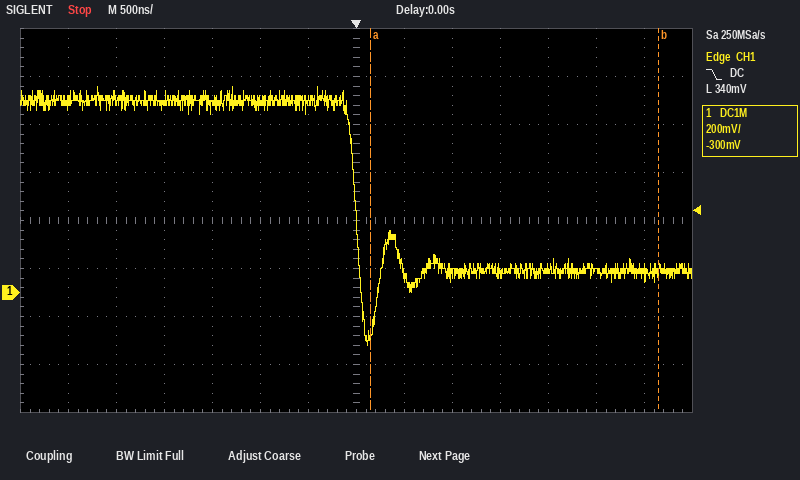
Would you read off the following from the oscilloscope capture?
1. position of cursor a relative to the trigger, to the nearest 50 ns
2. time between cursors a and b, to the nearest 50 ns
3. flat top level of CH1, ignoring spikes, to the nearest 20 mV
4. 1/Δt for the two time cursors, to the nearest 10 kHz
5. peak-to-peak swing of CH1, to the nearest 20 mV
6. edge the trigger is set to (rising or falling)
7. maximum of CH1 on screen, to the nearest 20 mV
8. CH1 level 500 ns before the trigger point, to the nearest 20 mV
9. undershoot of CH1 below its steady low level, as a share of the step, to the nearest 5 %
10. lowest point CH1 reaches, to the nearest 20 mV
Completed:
+150 ns
3.00 µs
800 mV
330 kHz
1.08 V
falling
860 mV
800 mV
45 %
-220 mV
